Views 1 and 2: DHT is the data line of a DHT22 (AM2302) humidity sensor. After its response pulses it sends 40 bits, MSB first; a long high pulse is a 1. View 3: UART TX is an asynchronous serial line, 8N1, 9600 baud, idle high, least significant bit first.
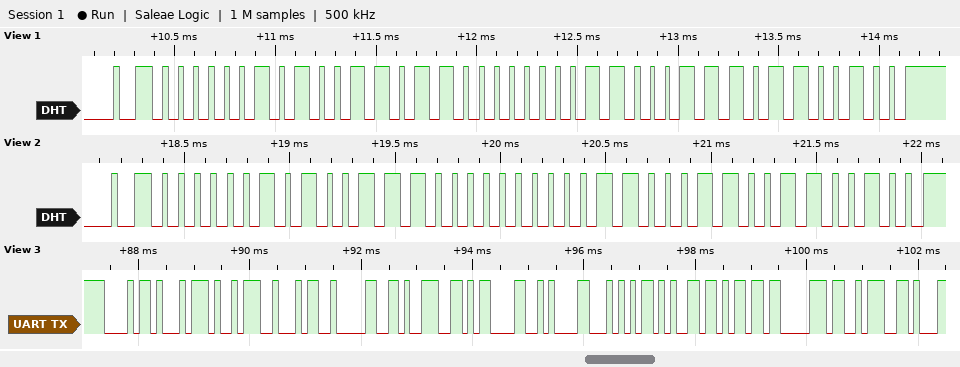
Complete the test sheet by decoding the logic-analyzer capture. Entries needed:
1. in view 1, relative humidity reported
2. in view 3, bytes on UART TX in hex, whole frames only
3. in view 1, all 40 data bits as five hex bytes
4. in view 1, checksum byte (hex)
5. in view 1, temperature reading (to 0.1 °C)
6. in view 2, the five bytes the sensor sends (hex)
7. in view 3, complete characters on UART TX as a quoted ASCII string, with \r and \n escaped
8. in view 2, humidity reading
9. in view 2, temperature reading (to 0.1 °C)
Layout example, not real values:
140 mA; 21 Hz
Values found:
66.7 %; 68 74 3A 34 30 39 0D 0A 54 65 6D 70 3A; 02 9B 00 C7 64; 0x64; 19.9 °C; 02 9C 00 C6 64; "ht:409\r\nTemp:"; 66.8 %; 19.8 °C
